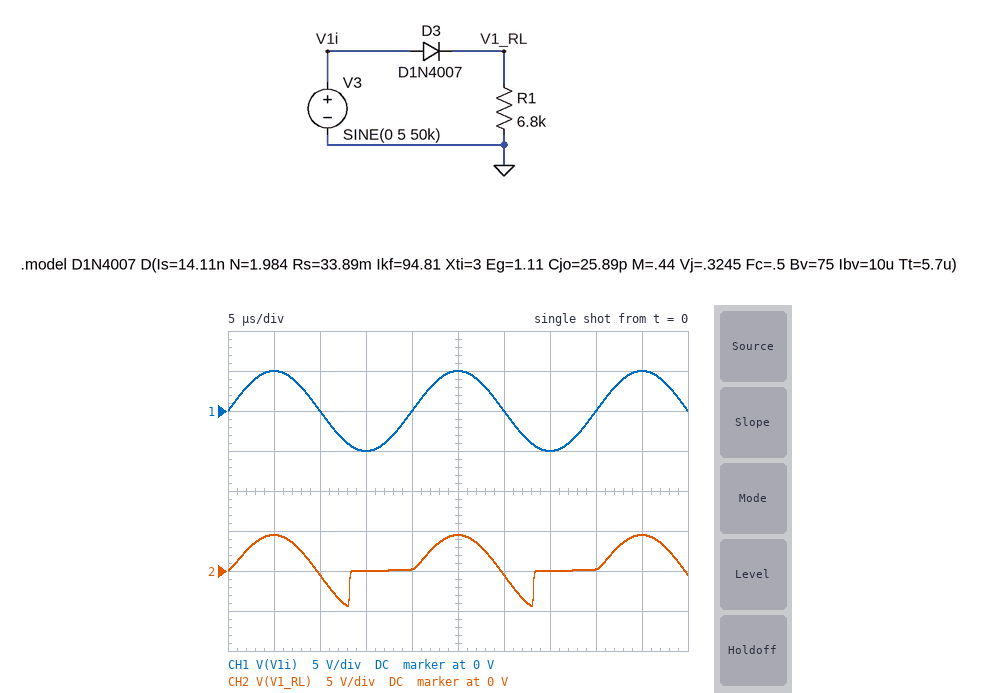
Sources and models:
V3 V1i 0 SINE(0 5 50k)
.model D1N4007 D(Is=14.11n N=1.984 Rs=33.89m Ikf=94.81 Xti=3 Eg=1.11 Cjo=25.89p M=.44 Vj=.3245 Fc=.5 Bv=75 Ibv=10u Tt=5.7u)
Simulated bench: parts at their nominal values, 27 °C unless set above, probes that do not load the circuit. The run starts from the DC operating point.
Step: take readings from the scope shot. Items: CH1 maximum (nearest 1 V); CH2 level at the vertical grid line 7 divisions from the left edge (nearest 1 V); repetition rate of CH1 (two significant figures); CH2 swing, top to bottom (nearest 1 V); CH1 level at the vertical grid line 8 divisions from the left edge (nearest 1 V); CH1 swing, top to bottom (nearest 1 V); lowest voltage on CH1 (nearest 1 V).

5 V
0 V
50 kHz
9 V
0 V
10 V
-5 V
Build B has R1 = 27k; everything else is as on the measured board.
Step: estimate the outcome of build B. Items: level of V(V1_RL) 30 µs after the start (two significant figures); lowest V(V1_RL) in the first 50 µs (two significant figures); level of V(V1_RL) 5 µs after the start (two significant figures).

-440 mV
-4.4 V
4.6 V
